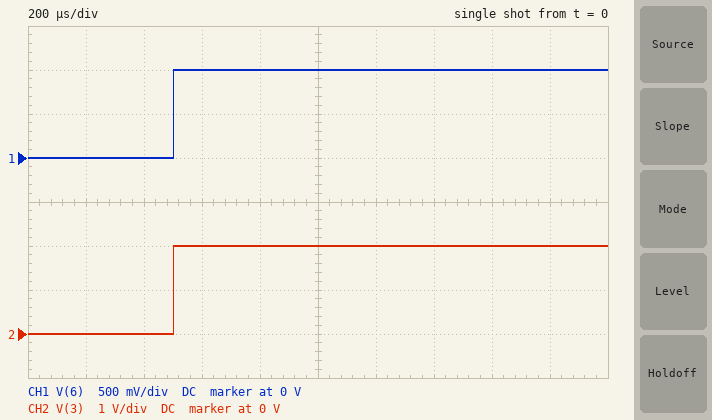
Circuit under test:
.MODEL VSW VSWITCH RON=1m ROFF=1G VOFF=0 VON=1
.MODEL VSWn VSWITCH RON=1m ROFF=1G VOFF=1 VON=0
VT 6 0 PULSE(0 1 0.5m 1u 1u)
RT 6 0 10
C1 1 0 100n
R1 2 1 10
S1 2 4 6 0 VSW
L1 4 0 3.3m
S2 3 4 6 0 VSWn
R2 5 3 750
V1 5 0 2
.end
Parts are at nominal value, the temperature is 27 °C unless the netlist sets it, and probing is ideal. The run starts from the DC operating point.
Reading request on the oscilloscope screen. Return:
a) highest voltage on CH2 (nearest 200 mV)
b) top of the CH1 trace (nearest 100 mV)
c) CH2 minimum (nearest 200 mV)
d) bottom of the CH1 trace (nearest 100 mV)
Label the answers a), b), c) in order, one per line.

a) 2.0 V
b) 1.0 V
c) 0 V
d) 0 V
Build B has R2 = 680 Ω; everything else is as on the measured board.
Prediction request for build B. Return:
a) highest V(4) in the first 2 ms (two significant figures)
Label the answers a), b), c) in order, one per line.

a) 470 mV
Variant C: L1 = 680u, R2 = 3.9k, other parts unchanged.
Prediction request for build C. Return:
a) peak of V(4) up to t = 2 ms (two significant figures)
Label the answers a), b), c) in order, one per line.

a) 31 mV
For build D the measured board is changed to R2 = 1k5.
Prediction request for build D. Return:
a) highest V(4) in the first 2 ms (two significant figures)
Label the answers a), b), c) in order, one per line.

a) 210 mV
